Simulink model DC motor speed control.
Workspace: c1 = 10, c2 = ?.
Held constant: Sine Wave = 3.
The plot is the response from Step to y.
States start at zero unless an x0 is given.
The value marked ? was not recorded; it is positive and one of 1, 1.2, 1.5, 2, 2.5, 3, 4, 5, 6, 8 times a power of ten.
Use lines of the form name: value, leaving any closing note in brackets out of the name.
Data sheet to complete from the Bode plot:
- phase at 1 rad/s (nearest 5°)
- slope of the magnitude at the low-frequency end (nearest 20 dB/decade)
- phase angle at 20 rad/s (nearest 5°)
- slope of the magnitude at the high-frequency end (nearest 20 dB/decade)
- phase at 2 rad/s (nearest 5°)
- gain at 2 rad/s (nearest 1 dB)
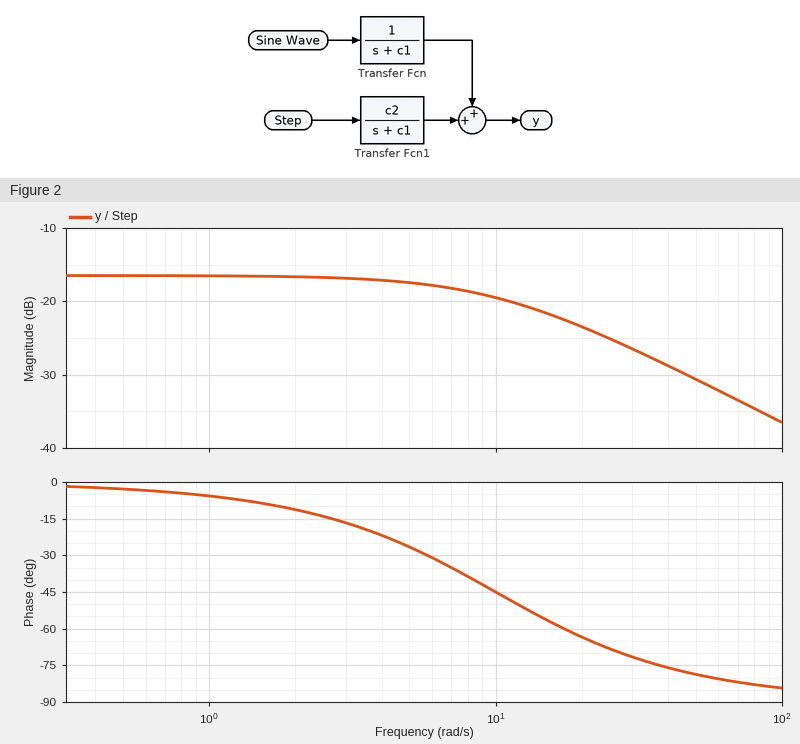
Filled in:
phase at 1 rad/s: -5°
slope of the magnitude at the low-frequency end: 0 dB/decade
phase angle at 20 rad/s: -65°
slope of the magnitude at the high-frequency end: -20 dB/decade
phase at 2 rad/s: -10°
gain at 2 rad/s: -17 dB
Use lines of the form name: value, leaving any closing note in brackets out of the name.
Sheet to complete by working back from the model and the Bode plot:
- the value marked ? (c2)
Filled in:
the value marked ?: 1.5
